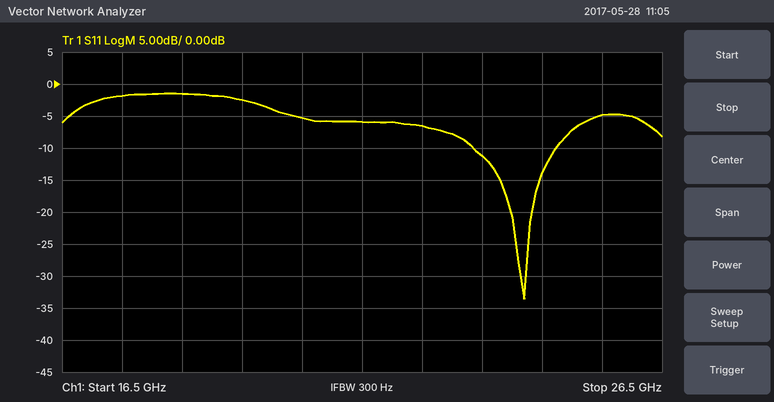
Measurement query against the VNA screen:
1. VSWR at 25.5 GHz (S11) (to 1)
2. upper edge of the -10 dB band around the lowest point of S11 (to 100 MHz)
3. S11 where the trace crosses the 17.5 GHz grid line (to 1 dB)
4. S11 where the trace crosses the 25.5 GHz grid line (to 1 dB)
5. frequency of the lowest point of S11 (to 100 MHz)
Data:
4
24.7 GHz
-2 dB
-5 dB
24.2 GHz
